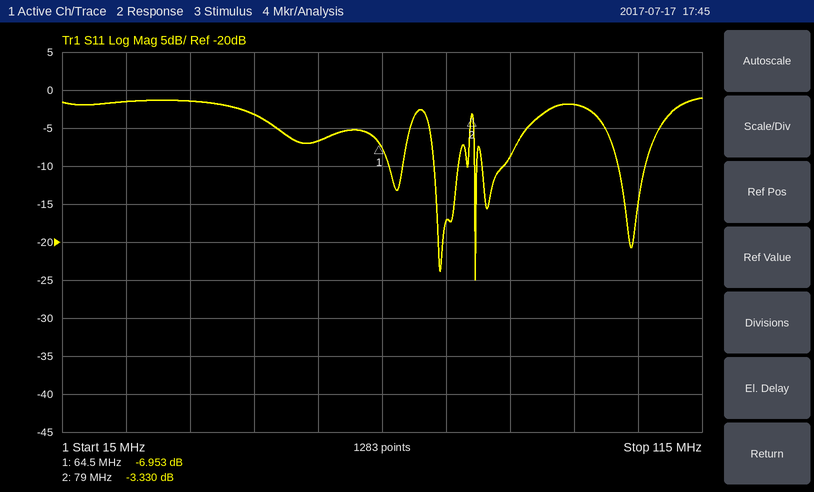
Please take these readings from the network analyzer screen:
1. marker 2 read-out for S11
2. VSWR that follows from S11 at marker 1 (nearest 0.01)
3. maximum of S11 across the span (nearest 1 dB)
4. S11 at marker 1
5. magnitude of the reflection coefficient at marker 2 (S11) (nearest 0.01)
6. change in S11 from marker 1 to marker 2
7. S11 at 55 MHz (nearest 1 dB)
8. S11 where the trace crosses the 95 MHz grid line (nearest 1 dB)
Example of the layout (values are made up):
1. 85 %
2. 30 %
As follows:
1. -3.330 dB
2. 2.63
3. -1 dB
4. -6.953 dB
5. 0.68
6. 3.623 dB
7. -7 dB
8. -2 dB
